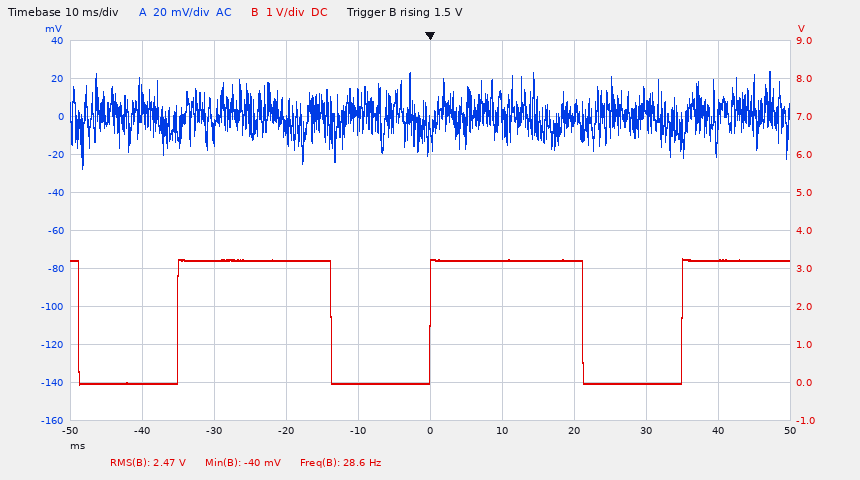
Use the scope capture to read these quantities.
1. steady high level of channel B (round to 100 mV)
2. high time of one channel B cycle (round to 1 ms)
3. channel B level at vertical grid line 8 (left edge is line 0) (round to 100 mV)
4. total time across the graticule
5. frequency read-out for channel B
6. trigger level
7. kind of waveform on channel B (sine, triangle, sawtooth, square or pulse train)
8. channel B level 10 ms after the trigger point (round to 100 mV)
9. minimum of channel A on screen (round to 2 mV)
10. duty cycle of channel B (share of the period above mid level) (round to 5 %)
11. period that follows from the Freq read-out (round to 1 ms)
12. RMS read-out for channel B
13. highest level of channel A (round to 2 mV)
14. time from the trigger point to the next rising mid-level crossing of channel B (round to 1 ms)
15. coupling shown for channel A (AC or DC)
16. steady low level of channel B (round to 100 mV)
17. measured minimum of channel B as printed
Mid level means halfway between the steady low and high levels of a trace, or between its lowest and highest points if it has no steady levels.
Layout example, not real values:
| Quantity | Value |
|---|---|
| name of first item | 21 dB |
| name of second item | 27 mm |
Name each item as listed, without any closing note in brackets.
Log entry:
| Quantity | Value |
|---|---|
| steady high level of channel B | 3.2 V |
| high time of one channel B cycle | 21 ms |
| channel B level at vertical grid line 8 (left edge is line 0) | 0.0 V |
| total time across the graticule | 100 ms |
| frequency read-out for channel B | 28.6 Hz |
| trigger level | 1.5 V |
| kind of waveform on channel B | pulse train |
| channel B level 10 ms after the trigger point | 3.2 V |
| minimum of channel A on screen | -28 mV |
| duty cycle of channel B (share of the period above mid level) | 60 % |
| period that follows from the Freq read-out | 35 ms |
| RMS read-out for channel B | 2.47 V |
| highest level of channel A | 24 mV |
| time from the trigger point to the next rising mid-level crossing of channel B | 35 ms |
| coupling shown for channel A | AC |
| steady low level of channel B | 0.0 V |
| measured minimum of channel B as printed | -40 mV |
